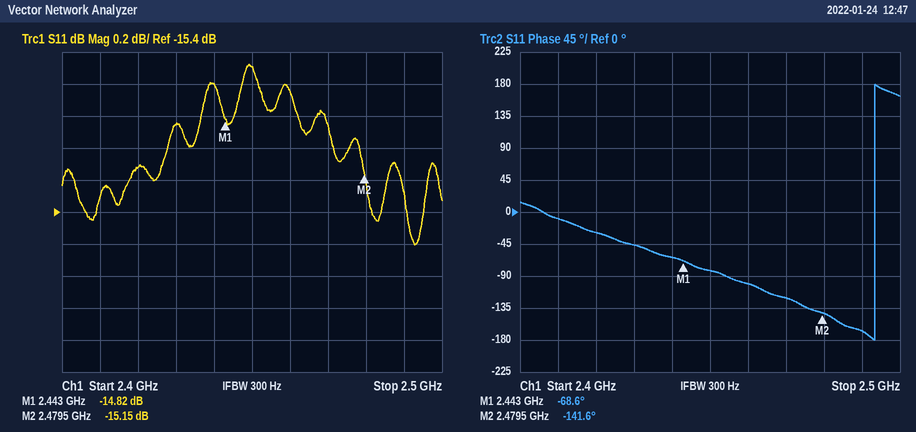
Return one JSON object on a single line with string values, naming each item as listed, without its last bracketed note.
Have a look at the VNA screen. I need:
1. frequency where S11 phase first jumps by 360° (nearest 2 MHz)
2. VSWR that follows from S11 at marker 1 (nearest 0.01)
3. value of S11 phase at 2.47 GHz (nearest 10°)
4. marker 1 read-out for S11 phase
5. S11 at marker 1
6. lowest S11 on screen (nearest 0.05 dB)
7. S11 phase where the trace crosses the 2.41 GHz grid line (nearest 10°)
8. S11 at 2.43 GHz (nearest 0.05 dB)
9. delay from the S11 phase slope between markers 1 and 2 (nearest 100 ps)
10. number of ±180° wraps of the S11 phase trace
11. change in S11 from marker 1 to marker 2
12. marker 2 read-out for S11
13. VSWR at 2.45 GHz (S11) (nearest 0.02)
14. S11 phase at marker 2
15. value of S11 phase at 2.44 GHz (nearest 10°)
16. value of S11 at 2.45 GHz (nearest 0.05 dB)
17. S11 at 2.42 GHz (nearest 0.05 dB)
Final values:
{"frequency where S11 phase first jumps by 360°": "2.494 GHz", "VSWR that follows from S11 at marker 1": "1.44", "value of S11 phase at 2.47 GHz": "-120°", "marker 1 read-out for S11 phase": "-68.6°", "S11 at marker 1": "-14.82 dB", "lowest S11 on screen": "-15.60 dB", "S11 phase where the trace crosses the 2.41 GHz grid line": "-10°", "S11 at 2.43 GHz": "-14.85 dB", "delay from the S11 phase slope between markers 1 and 2": "5.6 ns", "number of ±180° wraps of the S11 phase trace": "1", "change in S11 from marker 1 to marker 2": "-0.33 dB", "marker 2 read-out for S11": "-15.15 dB", "VSWR at 2.45 GHz (S11)": "1.46", "S11 phase at marker 2": "-141.6°", "value of S11 phase at 2.44 GHz": "-60°", "value of S11 at 2.45 GHz": "-14.50 dB", "S11 at 2.42 GHz": "-15.10 dB"}
